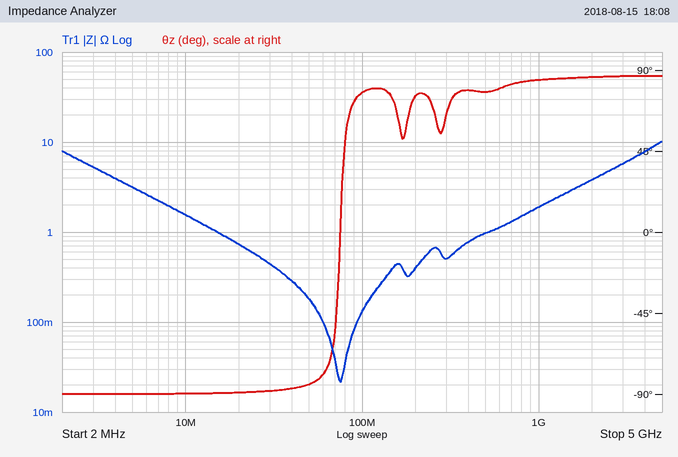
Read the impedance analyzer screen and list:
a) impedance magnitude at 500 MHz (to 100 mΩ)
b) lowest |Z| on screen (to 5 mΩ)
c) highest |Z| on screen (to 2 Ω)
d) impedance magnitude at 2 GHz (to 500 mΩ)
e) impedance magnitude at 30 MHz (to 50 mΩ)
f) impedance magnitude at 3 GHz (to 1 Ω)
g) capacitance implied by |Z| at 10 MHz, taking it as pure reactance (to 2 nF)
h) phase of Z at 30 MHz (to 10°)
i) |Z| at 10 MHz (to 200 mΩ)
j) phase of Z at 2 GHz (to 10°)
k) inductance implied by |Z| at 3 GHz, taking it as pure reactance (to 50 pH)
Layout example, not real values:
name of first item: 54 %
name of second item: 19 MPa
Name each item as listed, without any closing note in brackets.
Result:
impedance magnitude at 500 MHz: 1.0 Ω
lowest |Z| on screen: 20 mΩ
highest |Z| on screen: 10 Ω
impedance magnitude at 2 GHz: 4.0 Ω
impedance magnitude at 30 MHz: 450 mΩ
impedance magnitude at 3 GHz: 6 Ω
capacitance implied by |Z| at 10 MHz, taking it as pure reactance: 10 nF
phase of Z at 30 MHz: -90°
|Z| at 10 MHz: 1.6 Ω
phase of Z at 2 GHz: 90°
inductance implied by |Z| at 3 GHz, taking it as pure reactance: 300 pH
